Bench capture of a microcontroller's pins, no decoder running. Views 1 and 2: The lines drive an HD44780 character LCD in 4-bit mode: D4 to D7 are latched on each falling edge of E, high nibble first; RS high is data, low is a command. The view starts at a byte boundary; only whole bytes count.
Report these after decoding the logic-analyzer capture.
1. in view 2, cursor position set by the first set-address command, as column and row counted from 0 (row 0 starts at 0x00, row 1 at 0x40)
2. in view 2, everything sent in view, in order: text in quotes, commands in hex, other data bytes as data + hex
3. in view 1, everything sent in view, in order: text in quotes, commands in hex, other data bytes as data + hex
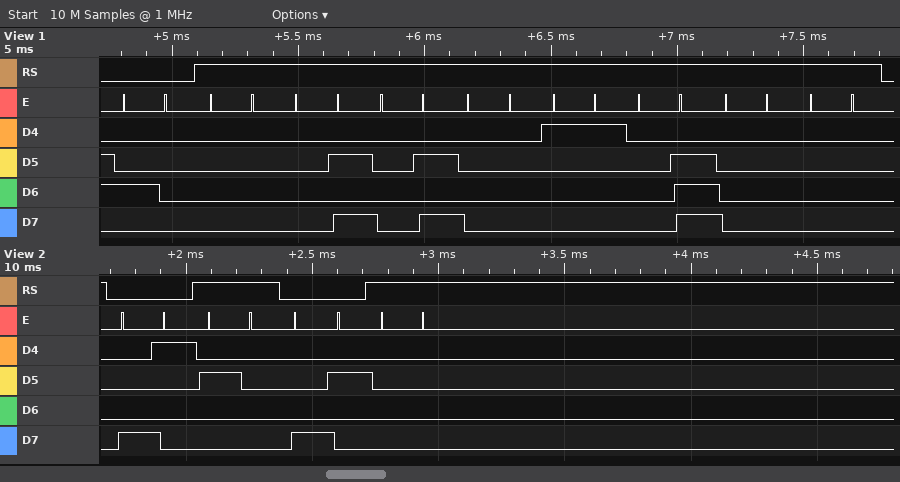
column 1, row 0
0x81 " " 0x82 data 00
0x40 data 00 0A 0A 00 11 0E 00 00
